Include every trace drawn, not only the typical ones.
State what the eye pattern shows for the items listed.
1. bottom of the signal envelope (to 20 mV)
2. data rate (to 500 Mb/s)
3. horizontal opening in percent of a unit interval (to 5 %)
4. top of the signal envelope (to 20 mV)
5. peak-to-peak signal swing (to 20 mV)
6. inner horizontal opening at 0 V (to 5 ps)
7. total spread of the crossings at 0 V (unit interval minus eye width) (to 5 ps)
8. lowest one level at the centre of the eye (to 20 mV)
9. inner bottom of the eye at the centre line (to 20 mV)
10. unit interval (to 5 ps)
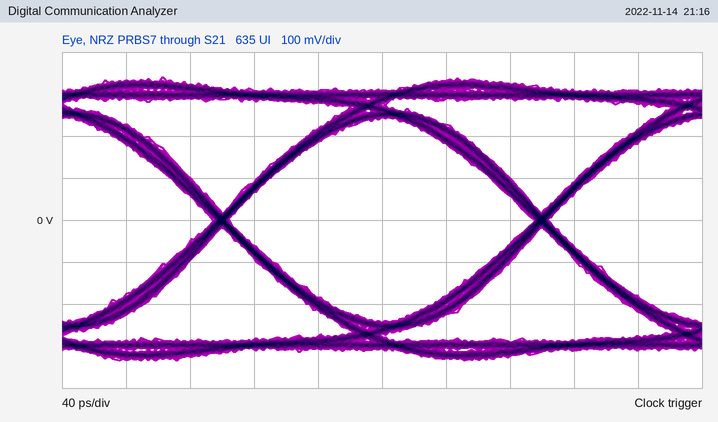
-340 mV
5.0 Gb/s
95 %
340 mV
680 mV
190 ps
10 ps
240 mV
-240 mV
200 ps
